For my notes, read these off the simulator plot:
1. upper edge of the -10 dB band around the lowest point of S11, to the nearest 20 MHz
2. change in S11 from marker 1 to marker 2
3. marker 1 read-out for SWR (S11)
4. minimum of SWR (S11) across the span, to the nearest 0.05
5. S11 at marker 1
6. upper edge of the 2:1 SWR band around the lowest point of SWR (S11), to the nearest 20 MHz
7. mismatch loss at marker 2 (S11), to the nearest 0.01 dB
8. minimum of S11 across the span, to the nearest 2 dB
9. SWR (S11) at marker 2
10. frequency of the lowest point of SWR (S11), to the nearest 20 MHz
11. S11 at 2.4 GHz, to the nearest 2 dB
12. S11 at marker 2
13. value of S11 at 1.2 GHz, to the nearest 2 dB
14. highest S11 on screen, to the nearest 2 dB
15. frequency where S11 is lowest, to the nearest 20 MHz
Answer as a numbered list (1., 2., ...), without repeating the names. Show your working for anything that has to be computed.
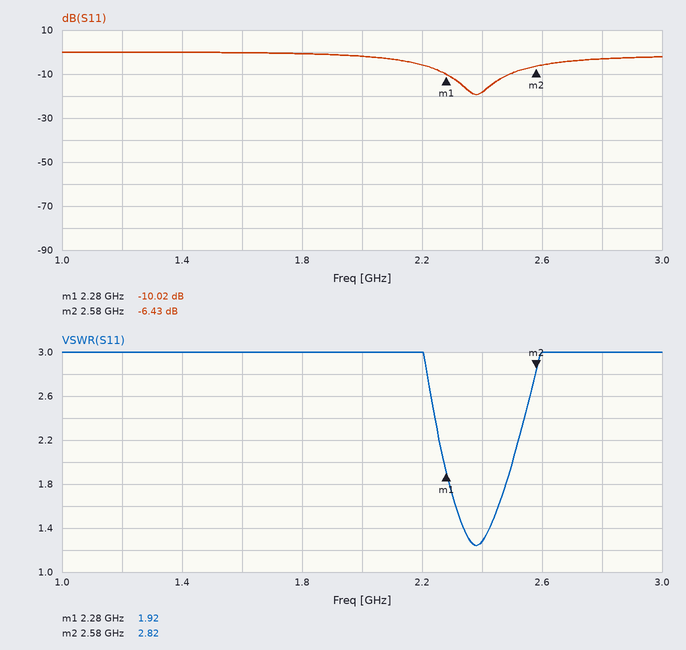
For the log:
1. 2.50 GHz
2. -6.43 − (-10.02) = 3.59 dB
3. 1.92
4. 1.25
5. -10.02 dB
6. 2.50 GHz
7. −10 log10(1 − 10^(-6.43/10)) ≈ 1.12 dB
8. -20 dB
9. 2.82
10. 2.38 GHz
11. -18 dB
12. -6.43 dB
13. 0 dB
14. 0 dB
15. 2.38 GHz
